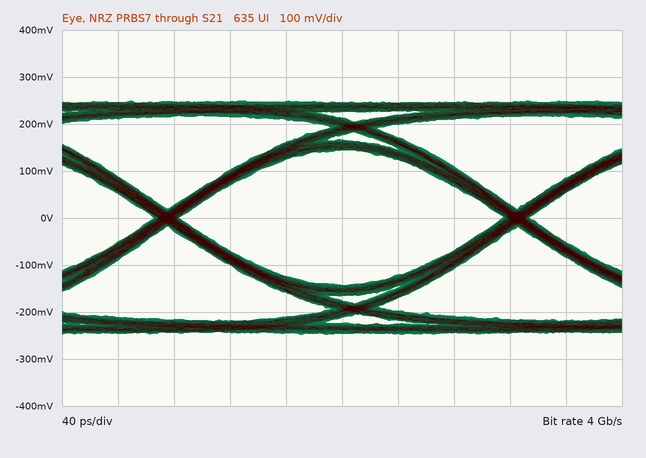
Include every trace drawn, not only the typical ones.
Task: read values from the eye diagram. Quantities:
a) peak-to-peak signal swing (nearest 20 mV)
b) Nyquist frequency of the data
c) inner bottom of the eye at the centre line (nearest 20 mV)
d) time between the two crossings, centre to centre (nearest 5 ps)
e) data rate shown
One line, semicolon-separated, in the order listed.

500 mV; 2 GHz; -140 mV; 250 ps; 4 Gb/s
